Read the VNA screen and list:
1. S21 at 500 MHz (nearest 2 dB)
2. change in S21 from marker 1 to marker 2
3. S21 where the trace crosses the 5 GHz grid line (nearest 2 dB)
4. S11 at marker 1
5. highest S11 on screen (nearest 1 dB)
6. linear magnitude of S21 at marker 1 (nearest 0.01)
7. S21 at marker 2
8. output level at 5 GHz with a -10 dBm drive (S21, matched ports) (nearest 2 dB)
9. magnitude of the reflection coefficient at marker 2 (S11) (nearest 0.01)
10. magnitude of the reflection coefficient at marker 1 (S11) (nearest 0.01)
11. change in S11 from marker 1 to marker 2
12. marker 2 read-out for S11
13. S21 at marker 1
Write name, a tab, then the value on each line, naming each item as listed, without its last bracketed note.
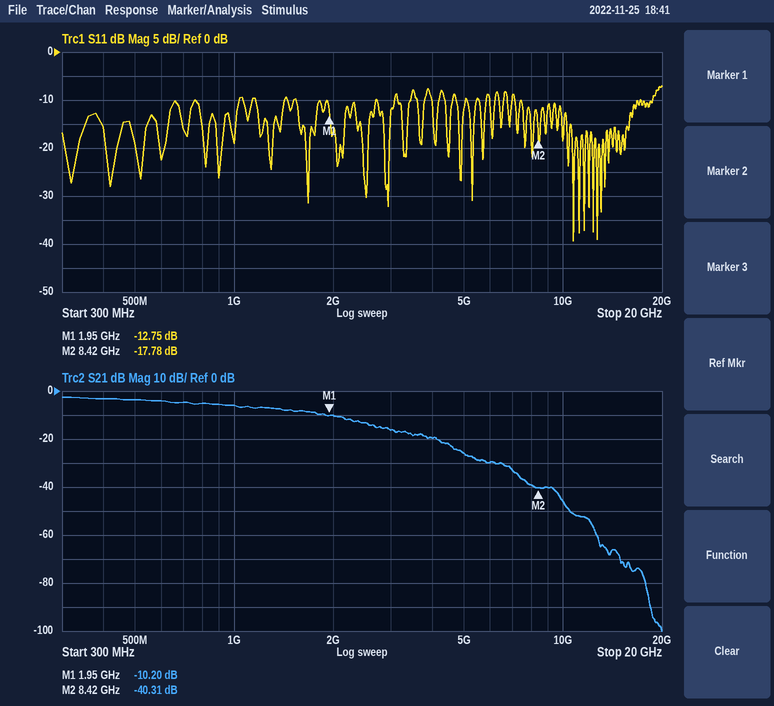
S21 at 500 MHz	-4 dB
change in S21 from marker 1 to marker 2	-30.11 dB
S21 where the trace crosses the 5 GHz grid line	-26 dB
S11 at marker 1	-12.75 dB
highest S11 on screen	-7 dB
linear magnitude of S21 at marker 1	0.31
S21 at marker 2	-40.31 dB
output level at 5 GHz with a -10 dBm drive (S21, matched ports)	-36 dBm
magnitude of the reflection coefficient at marker 2 (S11)	0.13
magnitude of the reflection coefficient at marker 1 (S11)	0.23
change in S11 from marker 1 to marker 2	-5.03 dB
marker 2 read-out for S11	-17.78 dB
S21 at marker 1	-10.20 dB
